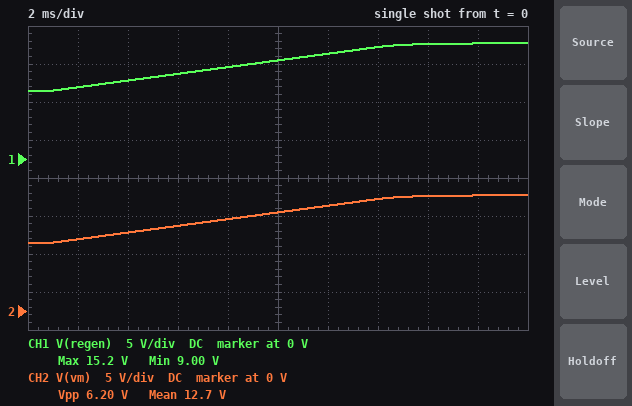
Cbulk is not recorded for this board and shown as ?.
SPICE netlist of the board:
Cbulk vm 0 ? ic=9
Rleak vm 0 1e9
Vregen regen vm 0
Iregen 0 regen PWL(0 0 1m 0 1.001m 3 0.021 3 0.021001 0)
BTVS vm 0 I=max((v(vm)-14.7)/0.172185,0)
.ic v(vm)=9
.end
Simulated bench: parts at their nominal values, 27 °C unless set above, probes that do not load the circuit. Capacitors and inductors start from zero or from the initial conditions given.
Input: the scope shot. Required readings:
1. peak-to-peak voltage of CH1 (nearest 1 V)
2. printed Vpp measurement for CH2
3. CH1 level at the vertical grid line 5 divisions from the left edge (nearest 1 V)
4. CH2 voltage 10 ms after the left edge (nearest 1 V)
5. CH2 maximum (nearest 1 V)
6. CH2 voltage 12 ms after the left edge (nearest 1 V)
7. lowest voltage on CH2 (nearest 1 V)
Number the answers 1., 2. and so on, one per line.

1. 6 V
2. 6.20 V
3. 13 V
4. 13 V
5. 15 V
6. 14 V
7. 9 V
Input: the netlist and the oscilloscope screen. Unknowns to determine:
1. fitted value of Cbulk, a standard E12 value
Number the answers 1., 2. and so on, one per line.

1. 6.8 mF
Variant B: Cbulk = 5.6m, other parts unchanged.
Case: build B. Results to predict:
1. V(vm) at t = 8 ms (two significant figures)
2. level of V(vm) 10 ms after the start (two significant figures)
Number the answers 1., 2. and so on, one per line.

1. 13 V
2. 14 V
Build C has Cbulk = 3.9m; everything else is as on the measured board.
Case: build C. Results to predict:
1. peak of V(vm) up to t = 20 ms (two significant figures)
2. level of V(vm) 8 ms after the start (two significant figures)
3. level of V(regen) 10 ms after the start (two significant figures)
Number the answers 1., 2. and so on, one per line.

1. 15 V
2. 14 V
3. 15 V
